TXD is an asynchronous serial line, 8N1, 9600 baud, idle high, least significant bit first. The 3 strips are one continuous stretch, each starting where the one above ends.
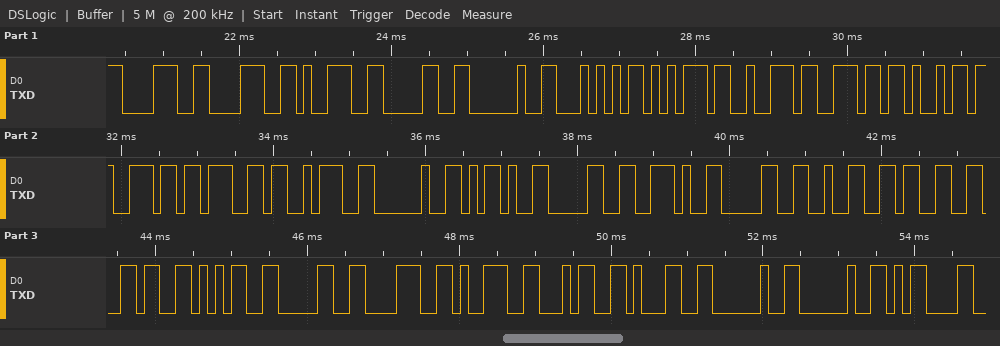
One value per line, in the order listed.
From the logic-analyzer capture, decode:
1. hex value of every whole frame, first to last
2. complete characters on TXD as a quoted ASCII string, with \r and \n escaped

38 38 39 30 20 54 75 72 6E 69 6E 67 3A 20 2D 30 2E 30 32 33 36 35 30 38 39 34 31 20 20 0D
"8890 Turning: -0.0236508941  \r"
